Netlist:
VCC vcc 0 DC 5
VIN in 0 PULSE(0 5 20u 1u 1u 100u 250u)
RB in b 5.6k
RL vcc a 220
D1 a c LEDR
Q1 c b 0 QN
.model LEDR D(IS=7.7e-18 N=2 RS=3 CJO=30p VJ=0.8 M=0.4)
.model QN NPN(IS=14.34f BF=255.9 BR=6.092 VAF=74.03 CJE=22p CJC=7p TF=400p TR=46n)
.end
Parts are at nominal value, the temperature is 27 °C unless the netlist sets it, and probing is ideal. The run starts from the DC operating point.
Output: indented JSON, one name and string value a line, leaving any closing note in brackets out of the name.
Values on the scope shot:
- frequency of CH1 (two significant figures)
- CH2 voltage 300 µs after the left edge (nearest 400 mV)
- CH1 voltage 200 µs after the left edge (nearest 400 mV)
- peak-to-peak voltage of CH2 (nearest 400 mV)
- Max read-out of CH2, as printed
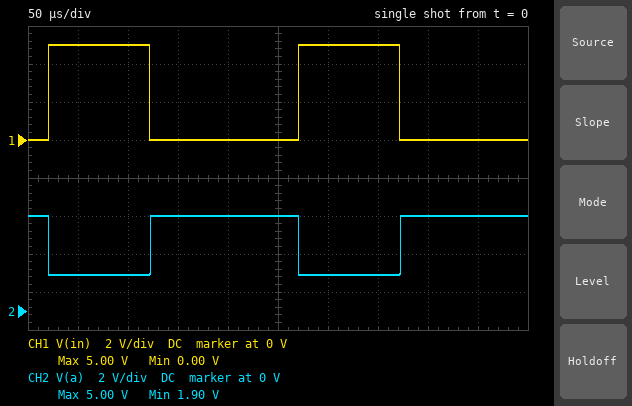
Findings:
{
  "frequency of CH1": "4.0 kHz",
  "CH2 voltage 300 µs after the left edge": "2.0 V",
  "CH1 voltage 200 µs after the left edge": "0 V",
  "peak-to-peak voltage of CH2": "3.2 V",
  "Max read-out of CH2, as printed": "5.00 V"
}
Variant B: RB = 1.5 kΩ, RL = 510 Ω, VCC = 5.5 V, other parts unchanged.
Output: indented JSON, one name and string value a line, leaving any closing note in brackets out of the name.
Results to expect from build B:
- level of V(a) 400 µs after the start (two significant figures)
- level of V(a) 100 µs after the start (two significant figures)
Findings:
{
  "level of V(a) 400 µs after the start": "5.5 V",
  "level of V(a) 100 µs after the start": "1.8 V"
}
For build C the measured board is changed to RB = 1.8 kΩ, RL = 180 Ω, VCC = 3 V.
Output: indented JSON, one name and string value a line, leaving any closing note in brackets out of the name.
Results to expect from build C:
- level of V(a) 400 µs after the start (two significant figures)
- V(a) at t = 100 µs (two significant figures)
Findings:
{
  "level of V(a) 400 µs after the start": "3.0 V",
  "V(a) at t = 100 µs": "1.8 V"
}
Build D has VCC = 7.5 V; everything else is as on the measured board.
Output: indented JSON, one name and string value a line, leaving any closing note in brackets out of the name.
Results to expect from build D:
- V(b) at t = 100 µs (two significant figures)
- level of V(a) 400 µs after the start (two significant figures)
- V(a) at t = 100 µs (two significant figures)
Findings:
{
  "V(b) at t = 100 µs": "730 mV",
  "level of V(a) 400 µs after the start": "7.5 V",
  "V(a) at t = 100 µs": "2.0 V"
}
